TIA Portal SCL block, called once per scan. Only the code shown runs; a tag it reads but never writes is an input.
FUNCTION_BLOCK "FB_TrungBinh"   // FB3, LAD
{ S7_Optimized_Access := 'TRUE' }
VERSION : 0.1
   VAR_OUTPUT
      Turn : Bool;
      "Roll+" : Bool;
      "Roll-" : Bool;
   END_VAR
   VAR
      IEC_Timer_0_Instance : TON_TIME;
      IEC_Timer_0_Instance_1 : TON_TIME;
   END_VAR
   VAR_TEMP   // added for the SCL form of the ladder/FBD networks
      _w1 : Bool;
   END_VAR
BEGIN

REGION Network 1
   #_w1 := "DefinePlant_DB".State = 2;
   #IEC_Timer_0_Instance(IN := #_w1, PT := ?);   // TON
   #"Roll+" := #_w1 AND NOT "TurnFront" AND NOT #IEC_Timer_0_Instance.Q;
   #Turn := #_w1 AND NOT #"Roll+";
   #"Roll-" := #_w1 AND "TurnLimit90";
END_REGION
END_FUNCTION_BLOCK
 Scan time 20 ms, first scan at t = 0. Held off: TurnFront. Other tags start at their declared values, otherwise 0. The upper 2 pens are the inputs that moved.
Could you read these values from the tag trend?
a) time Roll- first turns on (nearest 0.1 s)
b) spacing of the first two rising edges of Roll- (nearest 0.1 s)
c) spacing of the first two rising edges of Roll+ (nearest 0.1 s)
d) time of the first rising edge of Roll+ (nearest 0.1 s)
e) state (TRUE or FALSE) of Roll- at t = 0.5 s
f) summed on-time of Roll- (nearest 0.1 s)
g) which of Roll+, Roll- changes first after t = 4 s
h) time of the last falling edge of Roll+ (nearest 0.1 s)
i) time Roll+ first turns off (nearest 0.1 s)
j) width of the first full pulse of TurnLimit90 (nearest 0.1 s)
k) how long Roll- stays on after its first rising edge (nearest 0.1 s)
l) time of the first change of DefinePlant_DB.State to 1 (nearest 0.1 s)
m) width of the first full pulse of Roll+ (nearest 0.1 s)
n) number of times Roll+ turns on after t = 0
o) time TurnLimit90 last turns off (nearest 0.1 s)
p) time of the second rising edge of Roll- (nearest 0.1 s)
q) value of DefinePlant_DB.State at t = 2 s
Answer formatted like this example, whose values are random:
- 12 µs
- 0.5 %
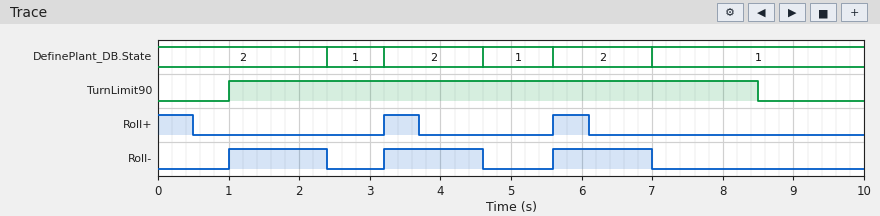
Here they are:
- 1.0 s
- 2.2 s
- 2.4 s
- 3.2 s
- FALSE
- 4.2 s
- Roll-
- 6.1 s
- 0.5 s
- 7.5 s
- 1.4 s
- 2.4 s
- 0.5 s
- 2
- 8.5 s
- 3.2 s
- 2
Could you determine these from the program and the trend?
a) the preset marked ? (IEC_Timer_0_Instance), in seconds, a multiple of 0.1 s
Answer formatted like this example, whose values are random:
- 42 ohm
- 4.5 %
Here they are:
- 0.5 s
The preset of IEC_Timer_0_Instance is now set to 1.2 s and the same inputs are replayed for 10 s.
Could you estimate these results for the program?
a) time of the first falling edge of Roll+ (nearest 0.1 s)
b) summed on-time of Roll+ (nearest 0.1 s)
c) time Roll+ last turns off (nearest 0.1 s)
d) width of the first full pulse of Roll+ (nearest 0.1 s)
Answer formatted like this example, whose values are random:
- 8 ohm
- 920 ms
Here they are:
- 1.2 s
- 3.6 s
- 6.8 s
- 1.2 s
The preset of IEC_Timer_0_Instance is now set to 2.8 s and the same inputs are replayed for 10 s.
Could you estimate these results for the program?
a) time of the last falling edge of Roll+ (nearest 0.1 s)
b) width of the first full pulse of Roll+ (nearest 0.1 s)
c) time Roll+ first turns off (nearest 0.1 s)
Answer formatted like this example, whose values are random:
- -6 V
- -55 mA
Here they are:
- 7.0 s
- 1.4 s
- 2.4 s
